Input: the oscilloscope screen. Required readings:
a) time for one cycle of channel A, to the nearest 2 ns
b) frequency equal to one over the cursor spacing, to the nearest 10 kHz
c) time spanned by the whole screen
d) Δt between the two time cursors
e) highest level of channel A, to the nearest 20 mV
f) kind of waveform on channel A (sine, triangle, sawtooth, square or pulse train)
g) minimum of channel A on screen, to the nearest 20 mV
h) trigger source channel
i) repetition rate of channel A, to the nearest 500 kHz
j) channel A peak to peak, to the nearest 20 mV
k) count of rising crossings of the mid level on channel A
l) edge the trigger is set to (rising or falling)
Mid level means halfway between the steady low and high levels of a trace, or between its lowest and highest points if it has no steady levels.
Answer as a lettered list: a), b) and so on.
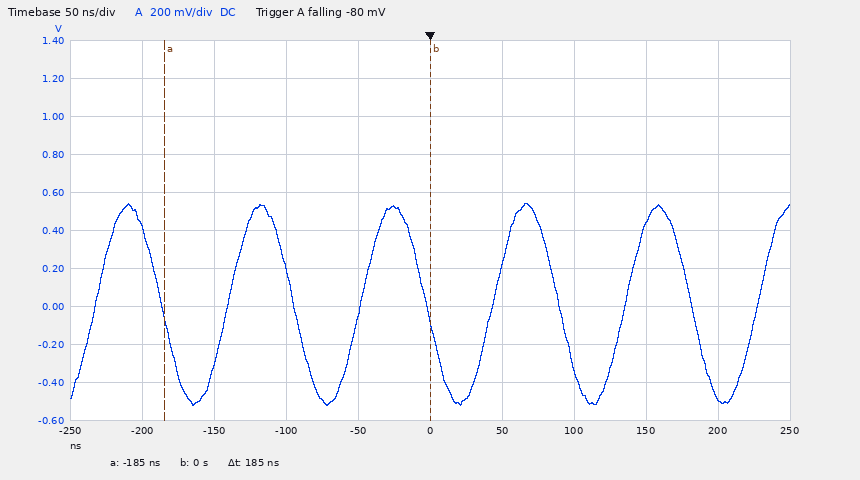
a) 92 ns
b) 5.41 MHz
c) 500 ns
d) 185 ns
e) 540 mV
f) sine
g) -520 mV
h) channel A
i) 11.0 MHz
j) 1.06 V
k) 6
l) falling
